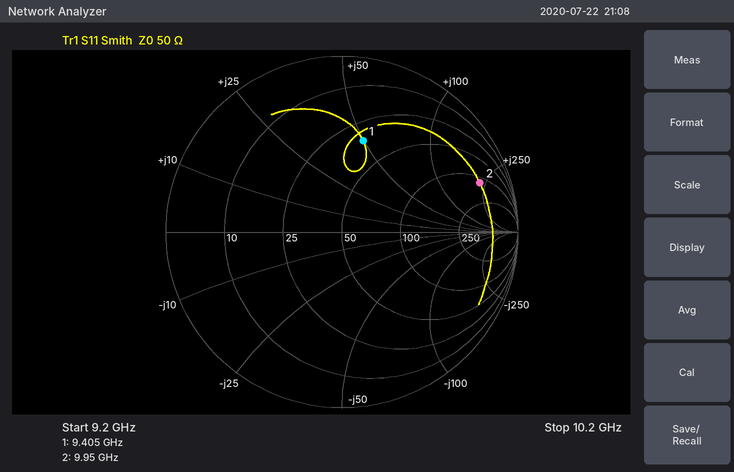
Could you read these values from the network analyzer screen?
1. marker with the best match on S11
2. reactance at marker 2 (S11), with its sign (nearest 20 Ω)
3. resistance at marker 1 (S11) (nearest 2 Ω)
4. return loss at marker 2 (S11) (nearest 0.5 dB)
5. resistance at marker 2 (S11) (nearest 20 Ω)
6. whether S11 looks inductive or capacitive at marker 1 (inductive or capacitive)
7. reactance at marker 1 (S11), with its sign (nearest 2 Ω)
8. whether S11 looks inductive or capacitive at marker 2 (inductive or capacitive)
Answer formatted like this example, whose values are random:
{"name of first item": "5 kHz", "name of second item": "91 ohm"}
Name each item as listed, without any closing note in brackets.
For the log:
{"marker with the best match on S11": "marker 1", "reactance at marker 2 (S11), with its sign": "+220 Ω", "resistance at marker 1 (S11)": "34 Ω", "return loss at marker 2 (S11)": "1.5 dB", "resistance at marker 2 (S11)": "120 Ω", "whether S11 looks inductive or capacitive at marker 1": "inductive", "reactance at marker 1 (S11), with its sign": "+50 Ω", "whether S11 looks inductive or capacitive at marker 2": "inductive"}
